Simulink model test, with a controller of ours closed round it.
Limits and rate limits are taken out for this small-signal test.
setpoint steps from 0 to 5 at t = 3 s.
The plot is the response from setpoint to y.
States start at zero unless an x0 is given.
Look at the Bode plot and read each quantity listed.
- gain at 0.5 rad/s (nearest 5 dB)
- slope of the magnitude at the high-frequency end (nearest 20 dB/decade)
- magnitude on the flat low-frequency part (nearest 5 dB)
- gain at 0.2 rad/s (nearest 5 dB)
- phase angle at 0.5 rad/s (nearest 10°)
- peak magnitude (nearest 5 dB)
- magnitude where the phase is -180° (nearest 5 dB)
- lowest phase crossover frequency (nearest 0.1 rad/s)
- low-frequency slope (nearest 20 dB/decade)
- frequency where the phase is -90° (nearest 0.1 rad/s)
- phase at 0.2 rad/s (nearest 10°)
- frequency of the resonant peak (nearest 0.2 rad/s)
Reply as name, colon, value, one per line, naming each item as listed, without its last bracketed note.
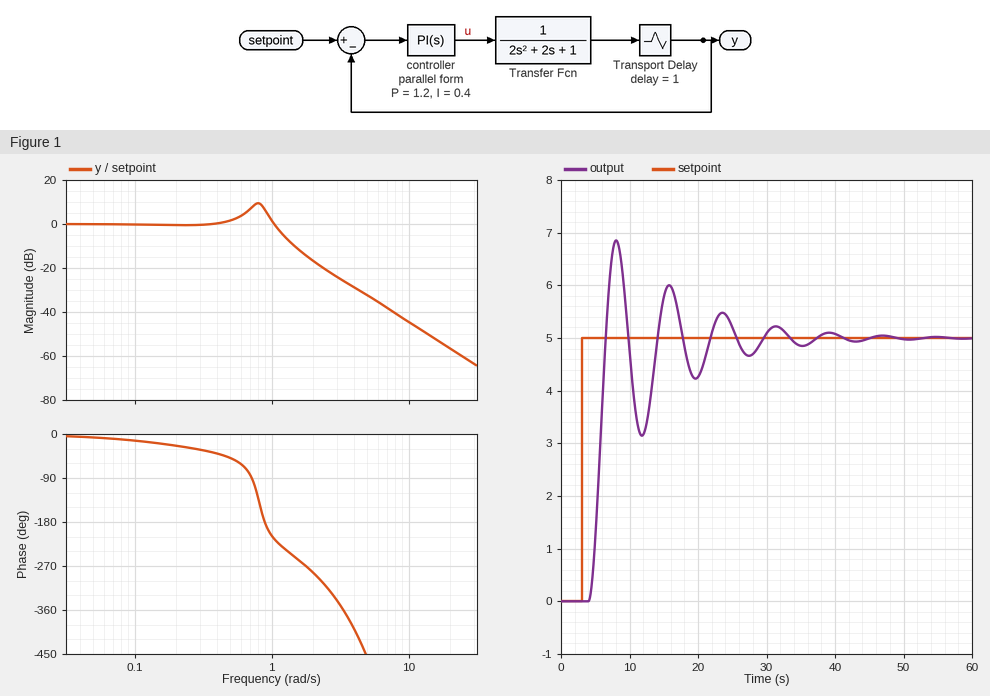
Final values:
gain at 0.5 rad/s: 0 dB
slope of the magnitude at the high-frequency end: -40 dB/decade
magnitude on the flat low-frequency part: 0 dB
gain at 0.2 rad/s: 0 dB
phase angle at 0.5 rad/s: -50°
peak magnitude: 10 dB
magnitude where the phase is -180°: 5 dB
lowest phase crossover frequency: 0.9 rad/s
low-frequency slope: 0 dB/decade
frequency where the phase is -90°: 0.7 rad/s
phase at 0.2 rad/s: -20°
frequency of the resonant peak: 0.8 rad/s
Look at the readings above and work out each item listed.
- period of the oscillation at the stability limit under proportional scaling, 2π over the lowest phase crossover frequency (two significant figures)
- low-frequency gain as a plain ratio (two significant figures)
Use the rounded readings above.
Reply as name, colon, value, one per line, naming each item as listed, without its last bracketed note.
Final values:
period of the oscillation at the stability limit under proportional scaling, 2π over the lowest phase crossover frequency: 7.0 s
low-frequency gain as a plain ratio: 1.0
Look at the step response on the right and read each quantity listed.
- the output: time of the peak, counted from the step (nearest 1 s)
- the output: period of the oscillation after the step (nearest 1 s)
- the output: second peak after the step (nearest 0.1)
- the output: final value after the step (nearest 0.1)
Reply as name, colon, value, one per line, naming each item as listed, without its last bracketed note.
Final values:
the output: time of the peak, counted from the step: 5 s
the output: period of the oscillation after the step: 8 s
the output: second peak after the step: 6.0
the output: final value after the step: 5.0
